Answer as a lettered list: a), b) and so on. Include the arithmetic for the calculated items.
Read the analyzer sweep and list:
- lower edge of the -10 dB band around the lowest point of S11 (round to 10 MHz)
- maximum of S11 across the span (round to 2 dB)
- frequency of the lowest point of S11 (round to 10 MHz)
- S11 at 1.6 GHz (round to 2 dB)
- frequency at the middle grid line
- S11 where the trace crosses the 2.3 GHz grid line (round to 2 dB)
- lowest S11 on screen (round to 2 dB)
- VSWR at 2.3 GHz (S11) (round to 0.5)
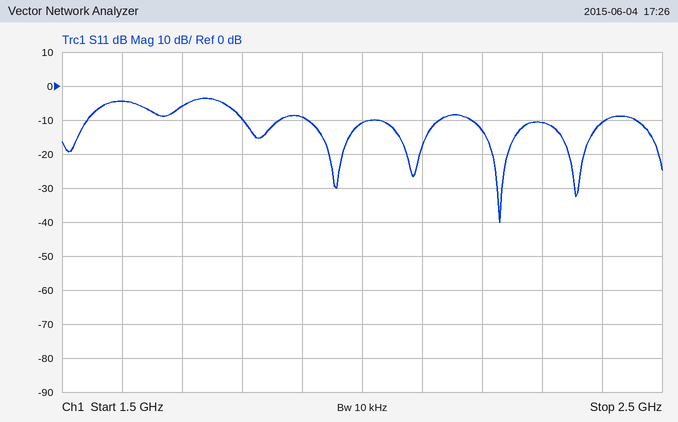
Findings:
a) 2.18 GHz
b) -4 dB
c) 2.23 GHz
d) -4 dB
e) 2 GHz
f) -10 dB
g) -40 dB
h) |Γ| = 10^(-10/20) = 0.3162; VSWR = (1 + 0.3162)/(1 − 0.3162) ≈ 1.92, so 2.0 to the nearest 0.5
